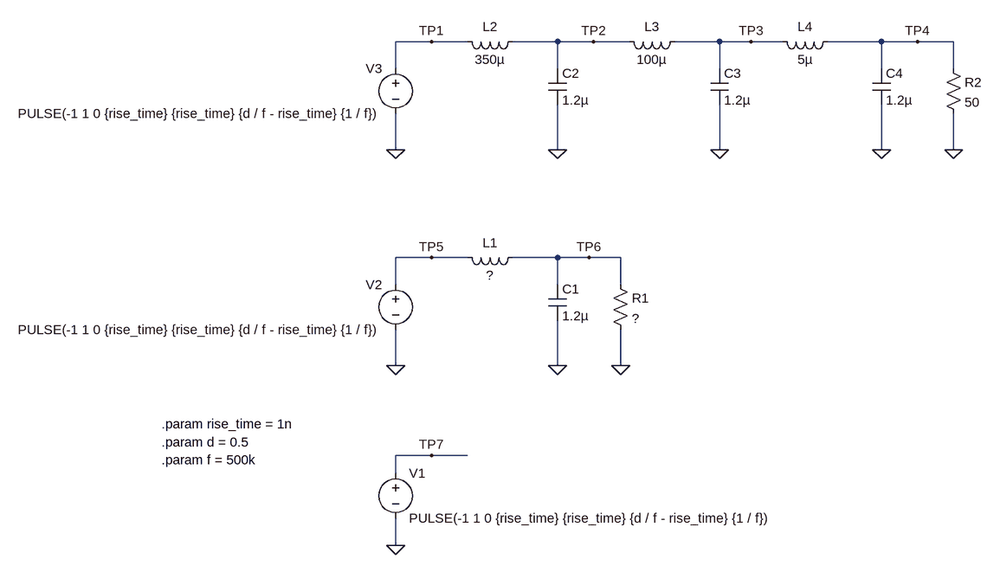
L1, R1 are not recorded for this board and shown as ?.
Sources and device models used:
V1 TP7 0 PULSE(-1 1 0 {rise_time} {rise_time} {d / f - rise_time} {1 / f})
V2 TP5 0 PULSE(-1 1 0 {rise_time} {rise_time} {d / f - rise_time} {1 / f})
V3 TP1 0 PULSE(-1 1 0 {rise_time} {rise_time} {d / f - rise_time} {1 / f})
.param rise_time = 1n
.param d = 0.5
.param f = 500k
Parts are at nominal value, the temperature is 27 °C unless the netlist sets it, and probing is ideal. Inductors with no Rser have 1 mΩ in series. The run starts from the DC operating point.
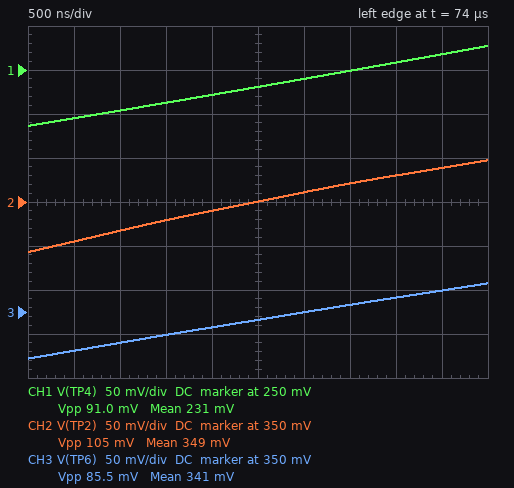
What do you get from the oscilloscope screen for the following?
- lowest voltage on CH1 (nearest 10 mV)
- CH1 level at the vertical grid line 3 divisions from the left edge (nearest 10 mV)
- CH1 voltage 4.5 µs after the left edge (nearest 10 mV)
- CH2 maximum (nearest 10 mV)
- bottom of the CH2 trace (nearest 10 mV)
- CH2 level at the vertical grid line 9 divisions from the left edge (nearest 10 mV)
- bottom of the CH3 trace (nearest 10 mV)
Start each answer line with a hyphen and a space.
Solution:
- 190 mV
- 210 mV
- 270 mV
- 400 mV
- 290 mV
- 390 mV
- 300 mV
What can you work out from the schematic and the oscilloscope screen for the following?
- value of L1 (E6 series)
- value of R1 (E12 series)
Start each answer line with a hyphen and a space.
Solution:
- 1 mH
- 100 Ω
